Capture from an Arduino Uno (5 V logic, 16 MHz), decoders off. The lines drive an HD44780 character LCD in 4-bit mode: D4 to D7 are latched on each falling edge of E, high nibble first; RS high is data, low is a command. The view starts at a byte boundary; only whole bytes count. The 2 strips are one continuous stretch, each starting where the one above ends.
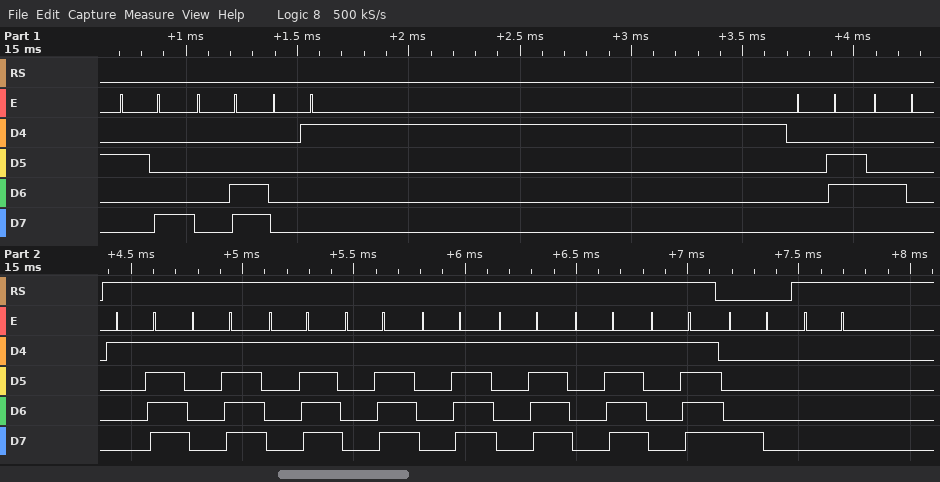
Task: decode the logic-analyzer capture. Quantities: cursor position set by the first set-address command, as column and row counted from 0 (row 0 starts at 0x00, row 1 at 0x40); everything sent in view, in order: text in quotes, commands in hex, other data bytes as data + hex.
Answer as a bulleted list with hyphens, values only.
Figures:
- column 0, row 0
- 0x28 0x0C 0x01 0x06 0x40 data 1F 1F 1F 1F 1F 1F 1F 1F 0x80 data 00
